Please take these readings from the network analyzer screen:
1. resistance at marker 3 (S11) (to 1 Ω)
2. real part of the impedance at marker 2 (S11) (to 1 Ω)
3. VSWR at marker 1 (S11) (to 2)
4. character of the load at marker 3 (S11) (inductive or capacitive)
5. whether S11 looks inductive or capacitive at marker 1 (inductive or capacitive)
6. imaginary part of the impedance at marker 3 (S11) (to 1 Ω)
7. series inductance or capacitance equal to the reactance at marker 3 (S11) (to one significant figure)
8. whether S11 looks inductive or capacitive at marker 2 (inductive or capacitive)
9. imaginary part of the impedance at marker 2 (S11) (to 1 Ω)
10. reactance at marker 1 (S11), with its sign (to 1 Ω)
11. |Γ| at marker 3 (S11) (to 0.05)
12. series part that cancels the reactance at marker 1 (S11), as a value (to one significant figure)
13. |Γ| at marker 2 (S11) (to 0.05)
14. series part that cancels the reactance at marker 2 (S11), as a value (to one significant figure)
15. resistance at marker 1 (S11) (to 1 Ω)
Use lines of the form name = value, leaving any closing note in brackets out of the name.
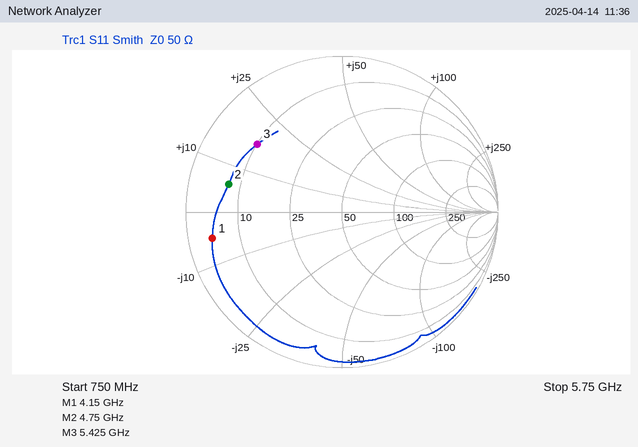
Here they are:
resistance at marker 3 (S11) = 10 Ω
real part of the impedance at marker 2 (S11) = 7 Ω
VSWR at marker 1 (S11) = 12
character of the load at marker 3 (S11) = inductive
whether S11 looks inductive or capacitive at marker 1 = capacitive
imaginary part of the impedance at marker 3 (S11) = +17 Ω
series inductance or capacitance equal to the reactance at marker 3 (S11) = 500 pH
whether S11 looks inductive or capacitive at marker 2 = inductive
imaginary part of the impedance at marker 2 (S11) = +6 Ω
reactance at marker 1 (S11), with its sign = -5 Ω
|Γ| at marker 3 (S11) = 0.70
series part that cancels the reactance at marker 1 (S11), as a value = 200 pH
|Γ| at marker 2 (S11) = 0.75
series part that cancels the reactance at marker 2 (S11), as a value = 6 pF
resistance at marker 1 (S11) = 4 Ω
